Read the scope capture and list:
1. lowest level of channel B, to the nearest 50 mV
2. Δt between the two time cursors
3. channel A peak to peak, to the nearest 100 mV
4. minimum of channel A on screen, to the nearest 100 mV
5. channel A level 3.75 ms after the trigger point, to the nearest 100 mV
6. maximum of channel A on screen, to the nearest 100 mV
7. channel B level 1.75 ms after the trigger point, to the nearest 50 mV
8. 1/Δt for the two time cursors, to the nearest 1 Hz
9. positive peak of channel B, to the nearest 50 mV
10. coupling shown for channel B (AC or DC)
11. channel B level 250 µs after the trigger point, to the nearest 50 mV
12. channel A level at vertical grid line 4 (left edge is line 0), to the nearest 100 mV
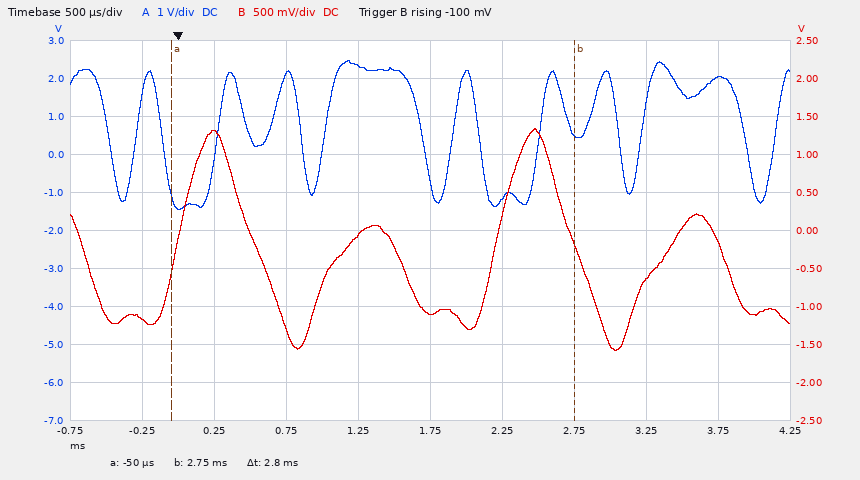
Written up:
-1.60 V
2.8 ms
3.9 V
-1.4 V
2.0 V
2.5 V
-1.10 V
357 Hz
1.35 V
DC
1.30 V
2.3 V
